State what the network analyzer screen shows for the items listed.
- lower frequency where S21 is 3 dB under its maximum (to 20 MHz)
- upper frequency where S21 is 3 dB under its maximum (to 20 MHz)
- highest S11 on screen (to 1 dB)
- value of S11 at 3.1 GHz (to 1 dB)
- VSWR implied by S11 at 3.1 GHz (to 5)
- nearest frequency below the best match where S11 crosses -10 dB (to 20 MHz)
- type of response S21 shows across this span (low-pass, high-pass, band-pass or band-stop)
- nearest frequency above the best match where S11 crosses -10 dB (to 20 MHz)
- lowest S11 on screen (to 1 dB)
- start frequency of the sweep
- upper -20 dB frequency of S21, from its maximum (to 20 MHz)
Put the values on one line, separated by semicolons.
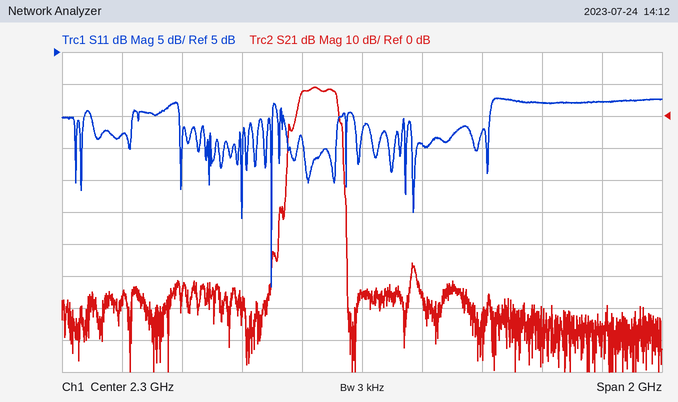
2.10 GHz; 2.22 GHz; -2 dB; -3 dB; 5; 2.00 GHz; band-pass; 2.00 GHz; -32 dB; 1.3 GHz; 2.24 GHz
